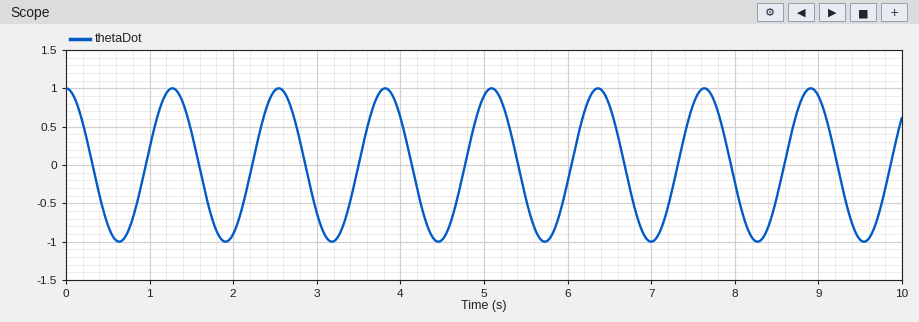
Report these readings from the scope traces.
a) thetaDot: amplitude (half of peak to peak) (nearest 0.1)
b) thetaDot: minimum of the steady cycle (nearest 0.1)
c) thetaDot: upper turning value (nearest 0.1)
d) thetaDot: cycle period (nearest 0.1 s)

1.0
-1.0
1.0
1.3 s
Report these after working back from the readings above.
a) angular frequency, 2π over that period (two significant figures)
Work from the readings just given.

4.8 rad/s
